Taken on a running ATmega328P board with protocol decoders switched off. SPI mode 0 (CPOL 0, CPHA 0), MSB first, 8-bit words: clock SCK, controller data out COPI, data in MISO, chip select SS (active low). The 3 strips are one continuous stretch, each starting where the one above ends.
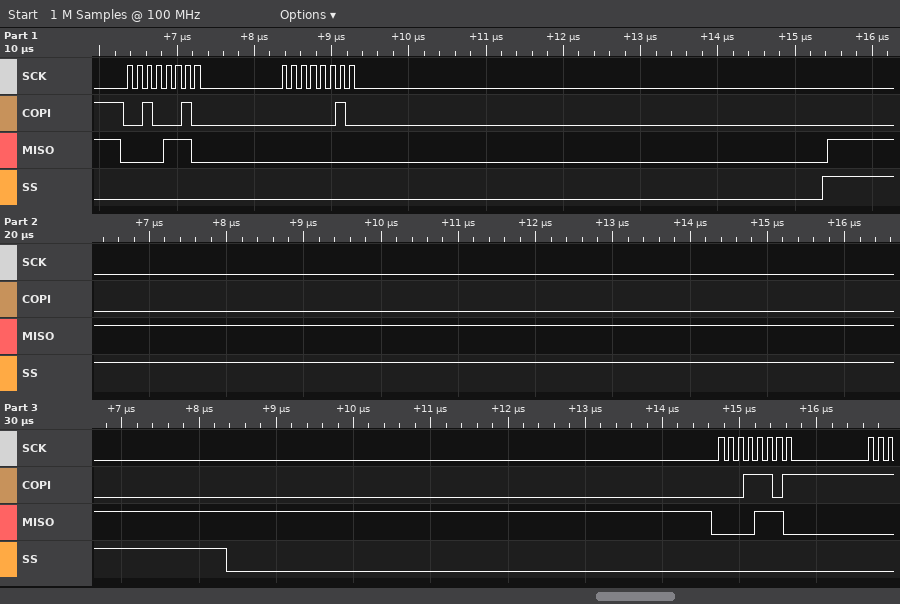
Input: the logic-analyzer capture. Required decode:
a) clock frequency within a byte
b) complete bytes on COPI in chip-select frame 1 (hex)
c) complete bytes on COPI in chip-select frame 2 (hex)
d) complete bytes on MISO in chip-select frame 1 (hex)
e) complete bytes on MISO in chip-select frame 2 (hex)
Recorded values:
8 MHz
22 02
1D
0E 00
0E
